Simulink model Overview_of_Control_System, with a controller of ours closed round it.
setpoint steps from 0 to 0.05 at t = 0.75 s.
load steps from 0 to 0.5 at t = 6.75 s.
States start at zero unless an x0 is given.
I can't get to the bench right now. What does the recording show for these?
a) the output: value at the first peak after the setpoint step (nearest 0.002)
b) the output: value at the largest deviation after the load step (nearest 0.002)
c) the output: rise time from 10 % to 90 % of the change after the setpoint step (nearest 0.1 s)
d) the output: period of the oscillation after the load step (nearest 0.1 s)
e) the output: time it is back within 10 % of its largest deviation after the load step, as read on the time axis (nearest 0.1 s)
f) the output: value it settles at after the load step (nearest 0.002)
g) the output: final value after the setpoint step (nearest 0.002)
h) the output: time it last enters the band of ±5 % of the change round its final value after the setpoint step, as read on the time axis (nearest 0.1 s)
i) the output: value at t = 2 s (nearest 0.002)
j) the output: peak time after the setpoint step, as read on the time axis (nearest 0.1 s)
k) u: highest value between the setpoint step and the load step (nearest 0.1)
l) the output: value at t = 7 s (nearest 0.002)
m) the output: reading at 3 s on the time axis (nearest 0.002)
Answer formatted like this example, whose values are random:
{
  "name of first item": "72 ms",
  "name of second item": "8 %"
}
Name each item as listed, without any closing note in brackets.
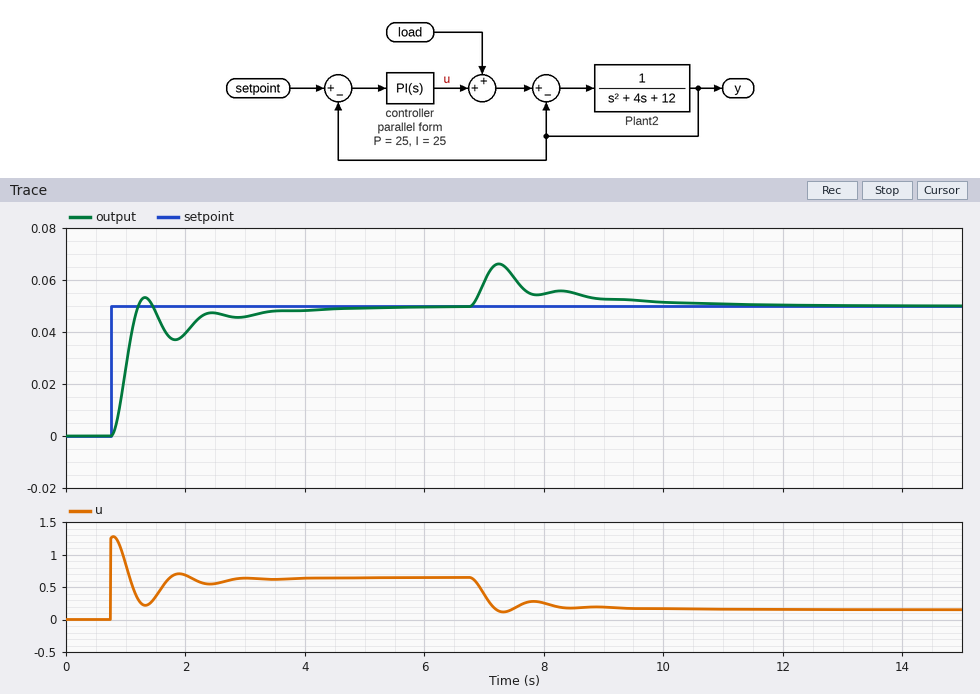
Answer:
{
  "the output: value at the first peak after the setpoint step": "0.054",
  "the output: value at the largest deviation after the load step": "0.066",
  "the output: rise time from 10 % to 90 % of the change after the setpoint step": "0.3 s",
  "the output: period of the oscillation after the load step": "1.0 s",
  "the output: time it is back within 10 % of its largest deviation after the load step, as read on the time axis": "9.8 s",
  "the output: value it settles at after the load step": "0.050",
  "the output: final value after the setpoint step": "0.050",
  "the output: time it last enters the band of ±5 % of the change round its final value after the setpoint step, as read on the time axis": "3.3 s",
  "the output: value at t = 2 s": "0.040",
  "the output: peak time after the setpoint step, as read on the time axis": "1.3 s",
  "u: highest value between the setpoint step and the load step": "1.3",
  "the output: value at t = 7 s": "0.060",
  "the output: reading at 3 s on the time axis": "0.046"
}
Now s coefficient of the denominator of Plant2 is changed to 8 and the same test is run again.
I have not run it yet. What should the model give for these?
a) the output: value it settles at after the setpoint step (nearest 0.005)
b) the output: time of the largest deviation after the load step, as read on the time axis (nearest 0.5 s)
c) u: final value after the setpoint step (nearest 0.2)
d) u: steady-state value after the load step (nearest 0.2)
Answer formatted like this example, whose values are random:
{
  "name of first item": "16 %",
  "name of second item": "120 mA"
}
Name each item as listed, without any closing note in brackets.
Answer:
{
  "the output: value it settles at after the setpoint step": "0.050",
  "the output: time of the largest deviation after the load step, as read on the time axis": "7.5 s",
  "u: final value after the setpoint step": "0.6",
  "u: steady-state value after the load step": "0.2"
}
